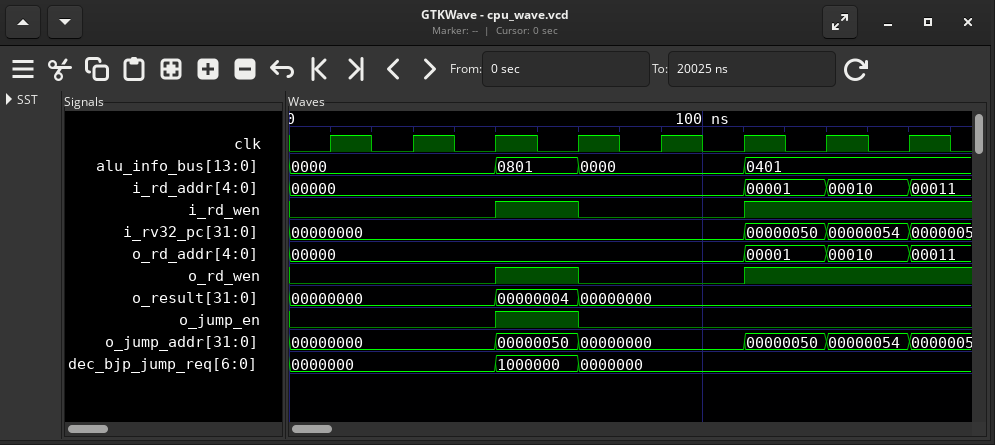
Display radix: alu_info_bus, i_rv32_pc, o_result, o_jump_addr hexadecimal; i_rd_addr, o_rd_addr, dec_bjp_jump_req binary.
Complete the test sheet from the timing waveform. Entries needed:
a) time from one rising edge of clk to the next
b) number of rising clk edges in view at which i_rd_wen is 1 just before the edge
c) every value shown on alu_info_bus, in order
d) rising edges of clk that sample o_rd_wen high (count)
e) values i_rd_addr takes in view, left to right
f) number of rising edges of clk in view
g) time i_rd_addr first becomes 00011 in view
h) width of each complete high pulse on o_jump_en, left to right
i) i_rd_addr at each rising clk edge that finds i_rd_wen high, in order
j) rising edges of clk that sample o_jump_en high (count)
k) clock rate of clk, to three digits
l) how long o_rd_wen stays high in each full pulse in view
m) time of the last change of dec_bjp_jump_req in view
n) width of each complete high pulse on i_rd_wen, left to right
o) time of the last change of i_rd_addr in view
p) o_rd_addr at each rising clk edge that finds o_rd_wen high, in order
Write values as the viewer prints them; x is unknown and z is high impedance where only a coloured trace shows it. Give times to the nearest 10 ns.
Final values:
20 ns
3
0000, 0801, 0000, 0401
3
00000, 00001, 00010, 00011
8
150 ns
20 ns
00000, 00001, 00010
1
50.0 MHz
20 ns
70 ns
20 ns
150 ns
00000, 00001, 00010
